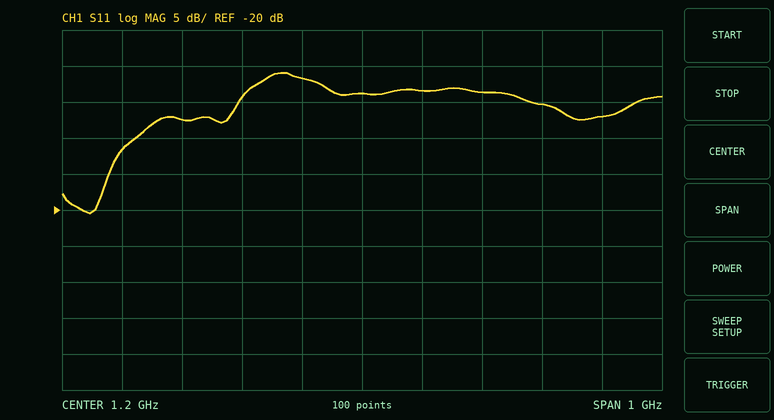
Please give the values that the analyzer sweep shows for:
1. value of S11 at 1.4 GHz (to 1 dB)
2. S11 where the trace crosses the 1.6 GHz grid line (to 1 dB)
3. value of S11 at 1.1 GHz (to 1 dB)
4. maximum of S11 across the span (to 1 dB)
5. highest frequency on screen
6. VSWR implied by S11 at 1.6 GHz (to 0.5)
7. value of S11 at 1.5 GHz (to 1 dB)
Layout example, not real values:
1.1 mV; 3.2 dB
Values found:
-4 dB; -7 dB; -2 dB; -1 dB; 1.7 GHz; 2.5; -5 dB
